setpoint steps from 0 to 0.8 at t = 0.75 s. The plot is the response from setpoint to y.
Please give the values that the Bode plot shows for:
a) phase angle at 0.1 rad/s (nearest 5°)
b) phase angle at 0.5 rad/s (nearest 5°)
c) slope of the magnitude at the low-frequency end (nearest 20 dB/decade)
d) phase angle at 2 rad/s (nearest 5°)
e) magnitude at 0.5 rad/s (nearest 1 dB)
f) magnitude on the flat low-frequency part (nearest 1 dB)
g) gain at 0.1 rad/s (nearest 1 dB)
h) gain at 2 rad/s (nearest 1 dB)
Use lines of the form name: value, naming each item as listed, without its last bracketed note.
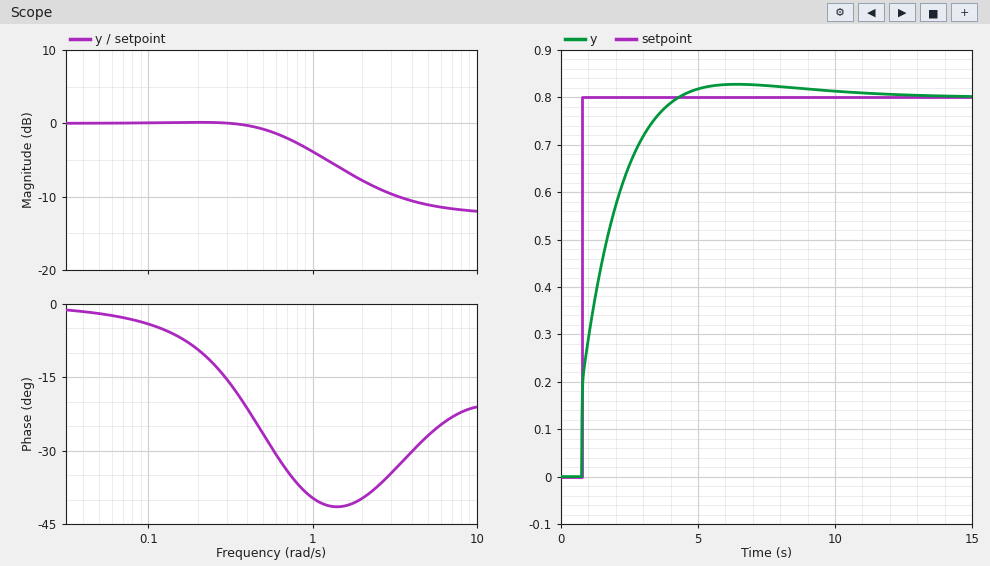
phase angle at 0.1 rad/s: -5°
phase angle at 0.5 rad/s: -25°
slope of the magnitude at the low-frequency end: 0 dB/decade
phase angle at 2 rad/s: -40°
magnitude at 0.5 rad/s: -1 dB
magnitude on the flat low-frequency part: 0 dB
gain at 0.1 rad/s: 0 dB
gain at 2 rad/s: -8 dB
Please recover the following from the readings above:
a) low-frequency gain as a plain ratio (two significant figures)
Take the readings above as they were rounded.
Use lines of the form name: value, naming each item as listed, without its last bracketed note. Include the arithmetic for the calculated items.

low-frequency gain as a plain ratio: 10^(0 / 20) = 1.0
